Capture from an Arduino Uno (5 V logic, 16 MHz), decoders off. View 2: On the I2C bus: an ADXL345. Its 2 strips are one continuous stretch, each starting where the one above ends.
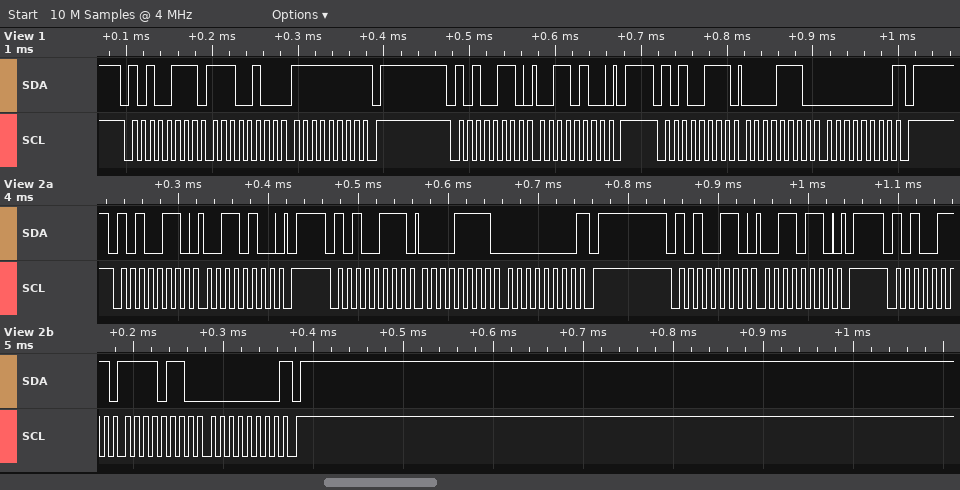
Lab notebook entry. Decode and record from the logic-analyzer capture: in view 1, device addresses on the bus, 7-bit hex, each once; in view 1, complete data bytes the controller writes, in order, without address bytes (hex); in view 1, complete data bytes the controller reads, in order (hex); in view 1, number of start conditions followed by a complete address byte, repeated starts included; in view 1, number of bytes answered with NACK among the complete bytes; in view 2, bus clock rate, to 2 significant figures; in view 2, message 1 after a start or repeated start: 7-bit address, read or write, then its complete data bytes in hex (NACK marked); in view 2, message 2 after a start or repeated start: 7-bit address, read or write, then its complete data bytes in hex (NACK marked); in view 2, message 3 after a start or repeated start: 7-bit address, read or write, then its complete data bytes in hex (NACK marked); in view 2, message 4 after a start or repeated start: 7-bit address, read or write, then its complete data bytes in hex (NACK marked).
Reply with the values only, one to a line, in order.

0x53
34
E4 FF 0E 00
3
2
100 kHz
0x53 write: 34
0x53 read: 0F 00 NACK
0x53 write: 36
0x53 read: F6 00 NACK
